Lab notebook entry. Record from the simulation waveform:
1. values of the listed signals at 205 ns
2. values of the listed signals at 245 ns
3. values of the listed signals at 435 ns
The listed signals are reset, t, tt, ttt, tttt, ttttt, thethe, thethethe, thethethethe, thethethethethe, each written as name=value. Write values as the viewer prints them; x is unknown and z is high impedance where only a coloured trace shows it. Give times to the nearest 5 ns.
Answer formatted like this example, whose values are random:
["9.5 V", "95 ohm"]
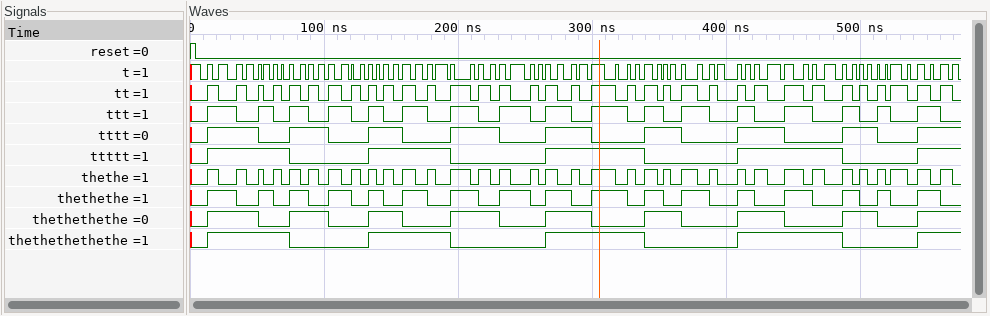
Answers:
["reset=0, t=0, tt=1, ttt=1, tttt=1, ttttt=0, thethe=1, thethethe=1, thethethethe=1, thethethethethe=0", "reset=0, t=1, tt=0, ttt=1, tttt=0, ttttt=0, thethe=0, thethethe=1, thethethethe=0, thethethethethe=0", "reset=0, t=1, tt=0, ttt=0, tttt=1, ttttt=1, thethe=0, thethethe=0, thethethethe=1, thethethethethe=1"]
